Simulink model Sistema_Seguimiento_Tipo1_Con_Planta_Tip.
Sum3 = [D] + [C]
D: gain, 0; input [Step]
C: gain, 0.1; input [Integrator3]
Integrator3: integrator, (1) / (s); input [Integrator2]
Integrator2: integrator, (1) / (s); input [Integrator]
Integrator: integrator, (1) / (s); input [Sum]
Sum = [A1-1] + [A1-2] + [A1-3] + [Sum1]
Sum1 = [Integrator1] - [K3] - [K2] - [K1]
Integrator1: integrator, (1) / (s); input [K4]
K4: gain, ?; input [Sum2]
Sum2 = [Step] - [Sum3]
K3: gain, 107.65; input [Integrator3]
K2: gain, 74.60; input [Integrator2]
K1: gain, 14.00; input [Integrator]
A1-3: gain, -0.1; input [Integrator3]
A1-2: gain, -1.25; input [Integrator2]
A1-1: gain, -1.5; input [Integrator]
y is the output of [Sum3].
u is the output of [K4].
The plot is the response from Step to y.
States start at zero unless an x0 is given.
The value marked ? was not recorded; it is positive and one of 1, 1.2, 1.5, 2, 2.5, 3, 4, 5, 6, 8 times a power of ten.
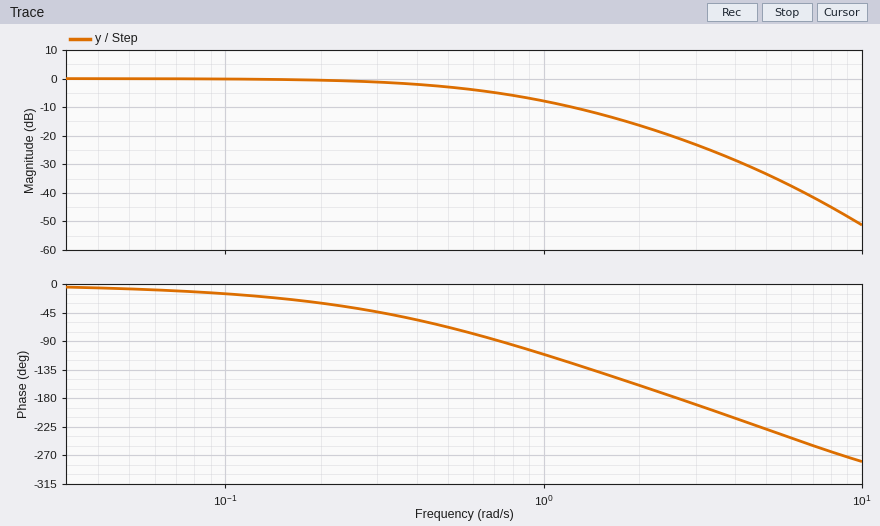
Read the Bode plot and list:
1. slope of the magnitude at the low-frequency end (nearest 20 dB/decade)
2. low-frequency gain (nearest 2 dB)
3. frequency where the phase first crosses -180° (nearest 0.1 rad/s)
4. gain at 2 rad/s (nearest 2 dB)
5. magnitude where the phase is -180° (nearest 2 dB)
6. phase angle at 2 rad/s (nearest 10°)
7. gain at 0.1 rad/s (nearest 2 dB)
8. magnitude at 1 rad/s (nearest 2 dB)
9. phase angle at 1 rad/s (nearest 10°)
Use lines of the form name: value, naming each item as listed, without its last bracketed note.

slope of the magnitude at the low-frequency end: 0 dB/decade
low-frequency gain: 0 dB
frequency where the phase first crosses -180°: 2.6 rad/s
gain at 2 rad/s: -16 dB
magnitude where the phase is -180°: -20 dB
phase angle at 2 rad/s: -160°
gain at 0.1 rad/s: 0 dB
magnitude at 1 rad/s: -8 dB
phase angle at 1 rad/s: -110°
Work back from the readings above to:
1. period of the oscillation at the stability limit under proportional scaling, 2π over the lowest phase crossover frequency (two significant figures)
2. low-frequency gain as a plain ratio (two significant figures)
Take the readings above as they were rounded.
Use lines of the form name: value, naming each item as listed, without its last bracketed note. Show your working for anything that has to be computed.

period of the oscillation at the stability limit under proportional scaling, 2π over the lowest phase crossover frequency: 2π / 2.6 = 2.4 s
low-frequency gain as a plain ratio: 10^(0 / 20) = 1.0
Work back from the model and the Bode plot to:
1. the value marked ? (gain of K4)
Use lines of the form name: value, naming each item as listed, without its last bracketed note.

the value marked ?: 400
